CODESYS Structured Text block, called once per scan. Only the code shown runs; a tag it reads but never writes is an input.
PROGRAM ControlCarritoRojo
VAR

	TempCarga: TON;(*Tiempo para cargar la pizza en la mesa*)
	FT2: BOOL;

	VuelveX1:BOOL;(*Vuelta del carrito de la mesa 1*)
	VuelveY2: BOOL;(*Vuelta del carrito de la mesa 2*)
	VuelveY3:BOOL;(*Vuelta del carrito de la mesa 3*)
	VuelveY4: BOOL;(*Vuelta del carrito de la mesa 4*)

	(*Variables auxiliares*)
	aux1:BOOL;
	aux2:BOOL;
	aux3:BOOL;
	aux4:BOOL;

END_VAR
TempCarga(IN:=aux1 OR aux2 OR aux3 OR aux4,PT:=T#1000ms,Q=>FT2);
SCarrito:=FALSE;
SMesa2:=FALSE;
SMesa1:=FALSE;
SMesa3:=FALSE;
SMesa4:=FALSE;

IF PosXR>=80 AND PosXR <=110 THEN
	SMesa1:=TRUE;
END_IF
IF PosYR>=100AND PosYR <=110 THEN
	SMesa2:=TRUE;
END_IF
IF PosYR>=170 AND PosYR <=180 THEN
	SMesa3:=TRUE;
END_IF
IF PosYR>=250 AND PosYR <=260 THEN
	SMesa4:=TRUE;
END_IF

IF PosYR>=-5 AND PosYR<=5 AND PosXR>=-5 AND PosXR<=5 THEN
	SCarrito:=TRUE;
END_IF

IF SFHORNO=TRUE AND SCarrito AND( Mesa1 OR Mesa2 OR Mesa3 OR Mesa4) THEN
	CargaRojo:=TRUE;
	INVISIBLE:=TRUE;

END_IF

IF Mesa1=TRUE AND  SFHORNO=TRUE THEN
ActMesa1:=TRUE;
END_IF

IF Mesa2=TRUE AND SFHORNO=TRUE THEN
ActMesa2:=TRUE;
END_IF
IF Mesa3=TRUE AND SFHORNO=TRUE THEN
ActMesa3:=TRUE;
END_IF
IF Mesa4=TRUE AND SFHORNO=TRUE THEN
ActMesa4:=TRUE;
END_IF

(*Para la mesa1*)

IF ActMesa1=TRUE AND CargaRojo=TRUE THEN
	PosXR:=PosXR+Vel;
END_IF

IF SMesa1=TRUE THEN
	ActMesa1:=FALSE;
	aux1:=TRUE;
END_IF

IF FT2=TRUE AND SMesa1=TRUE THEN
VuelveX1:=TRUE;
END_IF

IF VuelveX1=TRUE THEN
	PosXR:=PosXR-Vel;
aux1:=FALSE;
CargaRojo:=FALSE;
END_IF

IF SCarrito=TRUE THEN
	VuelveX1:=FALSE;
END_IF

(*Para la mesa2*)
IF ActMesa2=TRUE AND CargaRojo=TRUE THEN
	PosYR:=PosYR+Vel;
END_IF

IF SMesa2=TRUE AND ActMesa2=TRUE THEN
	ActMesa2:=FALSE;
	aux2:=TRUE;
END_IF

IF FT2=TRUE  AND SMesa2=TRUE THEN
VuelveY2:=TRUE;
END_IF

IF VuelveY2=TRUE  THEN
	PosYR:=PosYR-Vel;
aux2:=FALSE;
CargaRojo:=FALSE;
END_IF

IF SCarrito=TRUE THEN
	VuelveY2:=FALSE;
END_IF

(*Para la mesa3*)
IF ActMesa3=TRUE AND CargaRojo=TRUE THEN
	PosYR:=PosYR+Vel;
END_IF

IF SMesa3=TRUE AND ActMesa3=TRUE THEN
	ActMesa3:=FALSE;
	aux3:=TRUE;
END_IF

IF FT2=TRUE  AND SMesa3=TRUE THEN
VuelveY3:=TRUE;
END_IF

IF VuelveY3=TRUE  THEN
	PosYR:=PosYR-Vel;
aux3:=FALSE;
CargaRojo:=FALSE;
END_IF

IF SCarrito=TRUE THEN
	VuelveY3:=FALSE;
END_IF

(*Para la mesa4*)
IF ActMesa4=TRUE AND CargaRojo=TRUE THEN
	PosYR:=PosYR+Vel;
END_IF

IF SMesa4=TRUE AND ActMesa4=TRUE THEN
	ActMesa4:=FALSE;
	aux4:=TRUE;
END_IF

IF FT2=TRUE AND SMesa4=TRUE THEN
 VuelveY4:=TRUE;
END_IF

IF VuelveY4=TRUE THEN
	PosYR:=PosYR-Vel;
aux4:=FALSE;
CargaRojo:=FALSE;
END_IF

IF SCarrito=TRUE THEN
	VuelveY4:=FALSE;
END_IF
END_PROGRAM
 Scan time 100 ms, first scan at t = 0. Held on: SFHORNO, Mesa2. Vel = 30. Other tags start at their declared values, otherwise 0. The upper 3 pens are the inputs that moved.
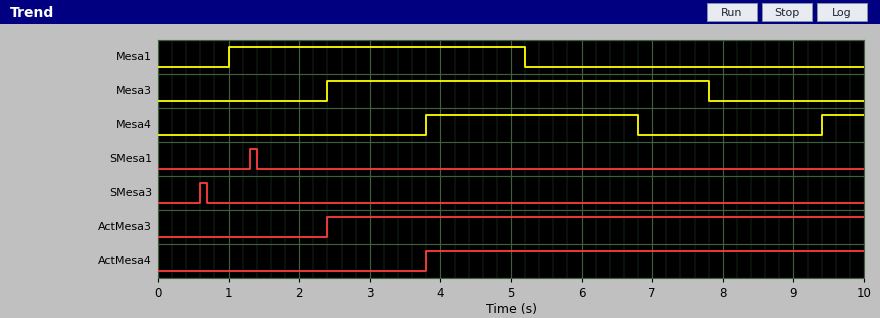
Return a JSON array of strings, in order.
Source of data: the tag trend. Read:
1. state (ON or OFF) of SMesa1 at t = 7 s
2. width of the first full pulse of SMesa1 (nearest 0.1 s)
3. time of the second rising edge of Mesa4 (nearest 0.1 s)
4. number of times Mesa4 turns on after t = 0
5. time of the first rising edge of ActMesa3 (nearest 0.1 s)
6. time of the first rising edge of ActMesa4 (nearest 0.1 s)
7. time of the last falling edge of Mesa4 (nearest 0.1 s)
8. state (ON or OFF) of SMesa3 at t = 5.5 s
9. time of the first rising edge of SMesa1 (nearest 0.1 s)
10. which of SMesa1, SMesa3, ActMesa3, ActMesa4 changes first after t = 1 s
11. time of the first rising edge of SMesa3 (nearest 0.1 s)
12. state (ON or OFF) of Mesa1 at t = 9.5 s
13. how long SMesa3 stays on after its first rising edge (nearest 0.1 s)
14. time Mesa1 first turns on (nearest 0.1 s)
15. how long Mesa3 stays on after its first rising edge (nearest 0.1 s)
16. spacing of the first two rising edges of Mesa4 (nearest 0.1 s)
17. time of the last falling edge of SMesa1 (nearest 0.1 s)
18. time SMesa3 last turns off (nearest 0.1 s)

["OFF", "0.1 s", "9.4 s", "2", "2.4 s", "3.8 s", "6.8 s", "OFF", "1.3 s", "SMesa1", "0.6 s", "OFF", "0.1 s", "1.0 s", "5.4 s", "5.6 s", "1.4 s", "0.7 s"]
